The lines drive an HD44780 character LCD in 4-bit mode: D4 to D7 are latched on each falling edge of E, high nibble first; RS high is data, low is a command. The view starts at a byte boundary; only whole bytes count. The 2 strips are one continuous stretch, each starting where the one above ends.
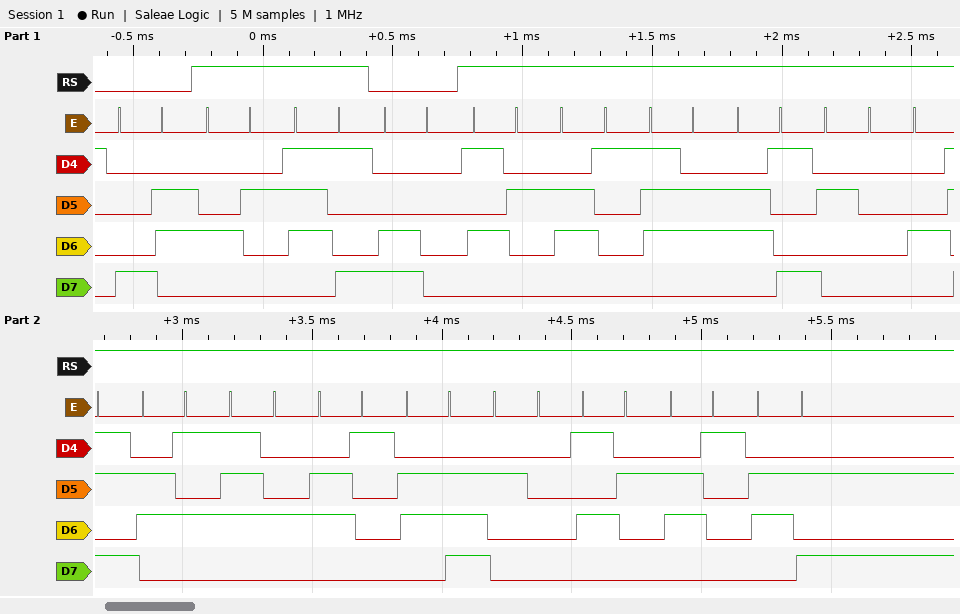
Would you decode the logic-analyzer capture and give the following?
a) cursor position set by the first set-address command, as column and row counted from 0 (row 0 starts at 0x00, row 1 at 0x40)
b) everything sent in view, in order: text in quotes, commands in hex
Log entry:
column 6, row 0
0x86 "By" 0xC0 "Ravi Ketan Raj"
